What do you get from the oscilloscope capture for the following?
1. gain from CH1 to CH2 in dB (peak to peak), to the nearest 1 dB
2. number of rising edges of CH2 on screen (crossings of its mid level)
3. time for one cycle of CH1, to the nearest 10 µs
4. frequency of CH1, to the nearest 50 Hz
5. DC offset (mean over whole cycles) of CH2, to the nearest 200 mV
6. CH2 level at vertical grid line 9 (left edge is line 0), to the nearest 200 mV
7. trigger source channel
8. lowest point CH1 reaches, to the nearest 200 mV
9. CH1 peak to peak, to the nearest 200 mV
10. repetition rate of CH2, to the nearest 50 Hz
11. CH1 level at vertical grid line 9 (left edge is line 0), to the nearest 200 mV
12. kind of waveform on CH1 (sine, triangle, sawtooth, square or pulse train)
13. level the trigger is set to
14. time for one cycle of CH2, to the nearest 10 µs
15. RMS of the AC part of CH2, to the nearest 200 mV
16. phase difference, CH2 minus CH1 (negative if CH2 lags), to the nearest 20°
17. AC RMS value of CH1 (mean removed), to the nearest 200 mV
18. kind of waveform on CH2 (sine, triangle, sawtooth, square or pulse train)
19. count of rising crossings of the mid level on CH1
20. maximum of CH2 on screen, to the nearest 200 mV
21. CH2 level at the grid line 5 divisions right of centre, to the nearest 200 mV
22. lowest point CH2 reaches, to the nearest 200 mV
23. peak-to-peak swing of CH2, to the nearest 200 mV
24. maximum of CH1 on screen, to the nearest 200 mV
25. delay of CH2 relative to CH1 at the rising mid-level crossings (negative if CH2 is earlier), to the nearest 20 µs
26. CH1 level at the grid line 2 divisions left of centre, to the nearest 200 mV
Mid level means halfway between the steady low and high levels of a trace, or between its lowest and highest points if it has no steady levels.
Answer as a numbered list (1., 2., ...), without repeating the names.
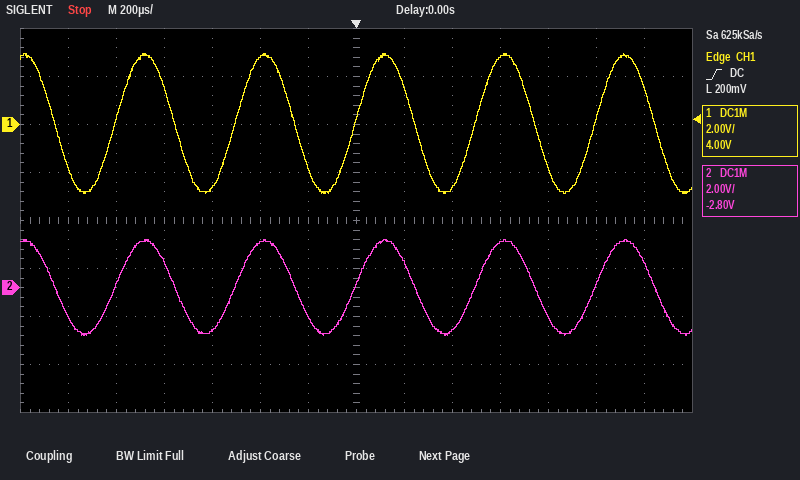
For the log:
1. -3 dB
2. 5
3. 500 µs
4. 2.00 kHz
5. 0.0 V
6. -1.8 V
7. CH1
8. -2.8 V
9. 5.8 V
10. 2.00 kHz
11. -2.6 V
12. sine
13. 200 mV
14. 500 µs
15. 1.4 V
16. 0°
17. 2.0 V
18. sine
19. 5
20. 2.0 V
21. 200 mV
22. -2.0 V
23. 4.0 V
24. 3.0 V
25. 0 µs
26. 2.8 V
